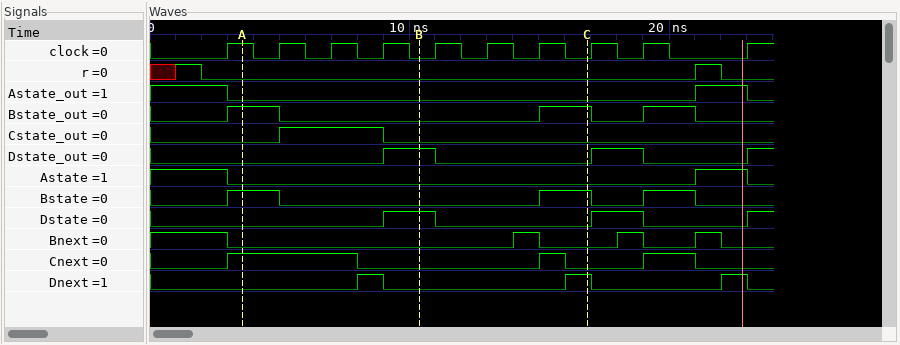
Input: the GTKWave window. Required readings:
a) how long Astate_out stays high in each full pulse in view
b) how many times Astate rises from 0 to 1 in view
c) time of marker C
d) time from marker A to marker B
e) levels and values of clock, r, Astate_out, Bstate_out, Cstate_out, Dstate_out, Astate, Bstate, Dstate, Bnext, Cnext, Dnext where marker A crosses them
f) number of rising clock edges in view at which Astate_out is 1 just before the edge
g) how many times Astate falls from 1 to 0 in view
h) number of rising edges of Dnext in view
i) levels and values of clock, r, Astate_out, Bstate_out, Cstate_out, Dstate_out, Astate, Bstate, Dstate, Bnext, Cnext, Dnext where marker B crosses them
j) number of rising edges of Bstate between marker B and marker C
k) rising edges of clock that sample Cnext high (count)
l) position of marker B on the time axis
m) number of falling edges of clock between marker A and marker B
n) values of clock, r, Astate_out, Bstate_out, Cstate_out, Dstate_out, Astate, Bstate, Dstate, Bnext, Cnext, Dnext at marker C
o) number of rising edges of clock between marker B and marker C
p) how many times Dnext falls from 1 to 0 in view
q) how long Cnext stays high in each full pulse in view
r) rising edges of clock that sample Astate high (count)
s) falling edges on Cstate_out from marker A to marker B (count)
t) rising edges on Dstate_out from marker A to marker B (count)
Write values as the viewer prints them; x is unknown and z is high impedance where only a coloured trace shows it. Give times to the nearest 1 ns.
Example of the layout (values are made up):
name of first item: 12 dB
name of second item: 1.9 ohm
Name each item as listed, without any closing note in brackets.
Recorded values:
how long Astate_out stays high in each full pulse in view: 2 ns
how many times Astate rises from 0 to 1 in view: 1
time of marker C: 17 ns
time from marker A to marker B: 7 ns
levels and values of clock, r, Astate_out, Bstate_out, Cstate_out, Dstate_out, Astate, Bstate, Dstate, Bnext, Cnext, Dnext where marker A crosses them: clock=1, r=0, Astate_out=0, Bstate_out=1, Cstate_out=0, Dstate_out=0, Astate=0, Bstate=1, Dstate=0, Bnext=0, Cnext=1, Dnext=0
number of rising clock edges in view at which Astate_out is 1 just before the edge: 2
how many times Astate falls from 1 to 0 in view: 2
number of rising edges of Dnext in view: 3
levels and values of clock, r, Astate_out, Bstate_out, Cstate_out, Dstate_out, Astate, Bstate, Dstate, Bnext, Cnext, Dnext where marker B crosses them: clock=0, r=0, Astate_out=0, Bstate_out=0, Cstate_out=0, Dstate_out=1, Astate=0, Bstate=0, Dstate=1, Bnext=0, Cnext=0, Dnext=0
number of rising edges of Bstate between marker B and marker C: 1
rising edges of clock that sample Cnext high: 2
position of marker B on the time axis: 10 ns
number of falling edges of clock between marker A and marker B: 4
values of clock, r, Astate_out, Bstate_out, Cstate_out, Dstate_out, Astate, Bstate, Dstate, Bnext, Cnext, Dnext at marker C: clock=0, r=0, Astate_out=0, Bstate_out=1, Cstate_out=0, Dstate_out=0, Astate=0, Bstate=1, Dstate=0, Bnext=0, Cnext=0, Dnext=1
number of rising edges of clock between marker B and marker C: 3
how many times Dnext falls from 1 to 0 in view: 3
how long Cnext stays high in each full pulse in view: 5 ns, 1 ns, 2 ns
rising edges of clock that sample Astate high: 2
falling edges on Cstate_out from marker A to marker B: 1
rising edges on Dstate_out from marker A to marker B: 1
